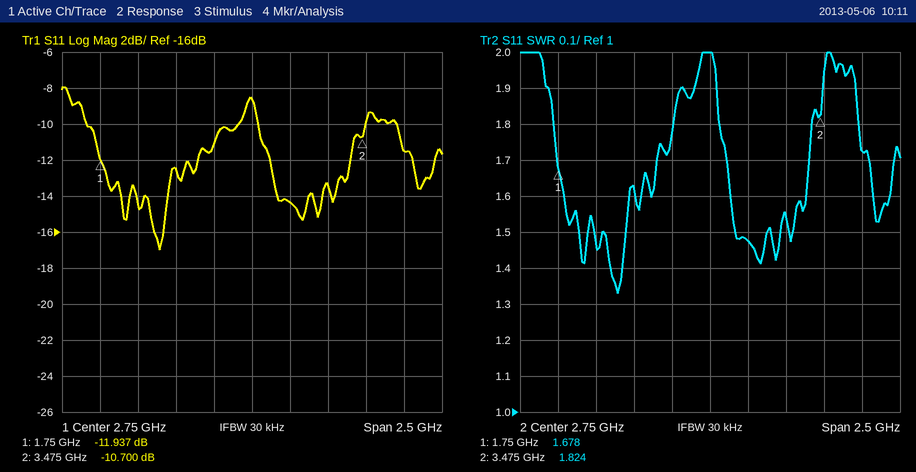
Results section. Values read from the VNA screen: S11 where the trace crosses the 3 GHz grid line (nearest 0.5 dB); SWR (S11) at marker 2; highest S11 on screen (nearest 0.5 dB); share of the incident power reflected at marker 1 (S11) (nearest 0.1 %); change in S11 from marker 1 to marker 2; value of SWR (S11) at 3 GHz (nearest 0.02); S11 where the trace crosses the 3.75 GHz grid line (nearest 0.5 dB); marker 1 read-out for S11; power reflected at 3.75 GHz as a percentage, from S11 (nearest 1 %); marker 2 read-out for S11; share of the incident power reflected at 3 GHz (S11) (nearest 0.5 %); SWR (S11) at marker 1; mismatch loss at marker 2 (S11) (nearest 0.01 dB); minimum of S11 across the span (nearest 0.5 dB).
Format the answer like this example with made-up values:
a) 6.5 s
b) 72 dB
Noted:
a) -14.5 dB
b) 1.824
c) -8.0 dB
d) 6.4 %
e) 1.237 dB
f) 1.48
g) -11.5 dB
h) -11.937 dB
i) 7 %
j) -10.700 dB
k) 3.5 %
l) 1.678
m) 0.39 dB
n) -17.0 dB
